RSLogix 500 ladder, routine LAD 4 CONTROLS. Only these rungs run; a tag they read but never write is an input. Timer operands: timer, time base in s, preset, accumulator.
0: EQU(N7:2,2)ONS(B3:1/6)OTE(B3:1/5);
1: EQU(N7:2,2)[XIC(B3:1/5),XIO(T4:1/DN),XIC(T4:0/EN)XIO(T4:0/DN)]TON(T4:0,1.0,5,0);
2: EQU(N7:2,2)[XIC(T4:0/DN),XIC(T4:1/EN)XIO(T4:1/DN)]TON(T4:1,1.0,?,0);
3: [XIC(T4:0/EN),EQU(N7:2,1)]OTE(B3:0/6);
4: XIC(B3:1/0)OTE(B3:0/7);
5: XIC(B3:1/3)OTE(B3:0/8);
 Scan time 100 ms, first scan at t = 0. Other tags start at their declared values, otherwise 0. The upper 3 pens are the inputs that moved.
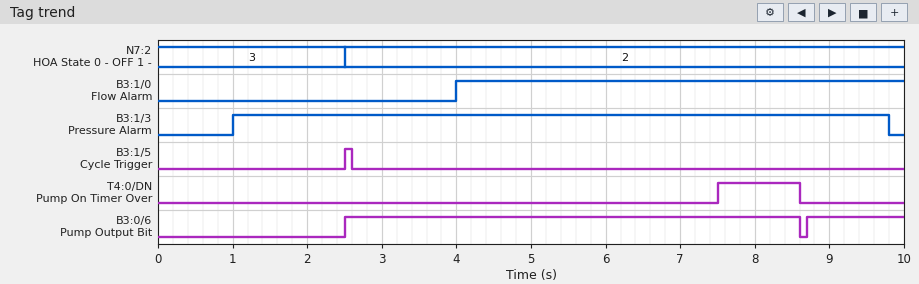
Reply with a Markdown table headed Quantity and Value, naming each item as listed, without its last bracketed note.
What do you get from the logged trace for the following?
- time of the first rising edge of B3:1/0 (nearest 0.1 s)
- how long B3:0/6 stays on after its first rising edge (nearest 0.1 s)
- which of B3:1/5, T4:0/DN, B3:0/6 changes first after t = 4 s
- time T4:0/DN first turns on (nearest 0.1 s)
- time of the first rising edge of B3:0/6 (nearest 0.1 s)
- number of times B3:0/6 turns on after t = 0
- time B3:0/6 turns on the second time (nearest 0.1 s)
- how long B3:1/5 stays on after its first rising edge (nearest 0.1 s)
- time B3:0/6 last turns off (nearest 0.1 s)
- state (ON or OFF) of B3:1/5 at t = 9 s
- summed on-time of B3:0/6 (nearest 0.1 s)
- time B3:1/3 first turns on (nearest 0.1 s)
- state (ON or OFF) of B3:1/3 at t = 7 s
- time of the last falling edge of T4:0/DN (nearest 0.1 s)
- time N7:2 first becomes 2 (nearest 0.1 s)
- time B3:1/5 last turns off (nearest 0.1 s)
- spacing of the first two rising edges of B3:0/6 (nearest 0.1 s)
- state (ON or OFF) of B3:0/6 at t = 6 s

| Quantity | Value |
|---|---|
| time of the first rising edge of B3:1/0 | 4.0 s |
| how long B3:0/6 stays on after its first rising edge | 6.1 s |
| which of B3:1/5, T4:0/DN, B3:0/6 changes first after t = 4 s | T4:0/DN |
| time T4:0/DN first turns on | 7.5 s |
| time of the first rising edge of B3:0/6 | 2.5 s |
| number of times B3:0/6 turns on after t = 0 | 2 |
| time B3:0/6 turns on the second time | 8.7 s |
| how long B3:1/5 stays on after its first rising edge | 0.1 s |
| time B3:0/6 last turns off | 8.6 s |
| state (ON or OFF) of B3:1/5 at t = 9 s | OFF |
| summed on-time of B3:0/6 | 7.4 s |
| time B3:1/3 first turns on | 1.0 s |
| state (ON or OFF) of B3:1/3 at t = 7 s | ON |
| time of the last falling edge of T4:0/DN | 8.6 s |
| time N7:2 first becomes 2 | 2.5 s |
| time B3:1/5 last turns off | 2.6 s |
| spacing of the first two rising edges of B3:0/6 | 6.2 s |
| state (ON or OFF) of B3:0/6 at t = 6 s | ON |
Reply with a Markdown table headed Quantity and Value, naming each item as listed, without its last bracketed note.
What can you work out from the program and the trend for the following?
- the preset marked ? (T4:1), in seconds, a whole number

| Quantity | Value |
|---|---|
| the preset marked ? (T4:1), in seconds, a whole number | 1 s |
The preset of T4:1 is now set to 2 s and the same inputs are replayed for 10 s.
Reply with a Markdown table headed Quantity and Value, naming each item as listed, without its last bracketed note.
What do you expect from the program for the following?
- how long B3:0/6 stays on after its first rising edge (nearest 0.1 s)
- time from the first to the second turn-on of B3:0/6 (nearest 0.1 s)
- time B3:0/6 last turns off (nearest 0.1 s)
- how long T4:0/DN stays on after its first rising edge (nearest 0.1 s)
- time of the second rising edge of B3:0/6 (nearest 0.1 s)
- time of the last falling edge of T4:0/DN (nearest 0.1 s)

| Quantity | Value |
|---|---|
| how long B3:0/6 stays on after its first rising edge | 7.1 s |
| time from the first to the second turn-on of B3:0/6 | 7.2 s |
| time B3:0/6 last turns off | 9.6 s |
| how long T4:0/DN stays on after its first rising edge | 2.1 s |
| time of the second rising edge of B3:0/6 | 9.7 s |
| time of the last falling edge of T4:0/DN | 9.6 s |
